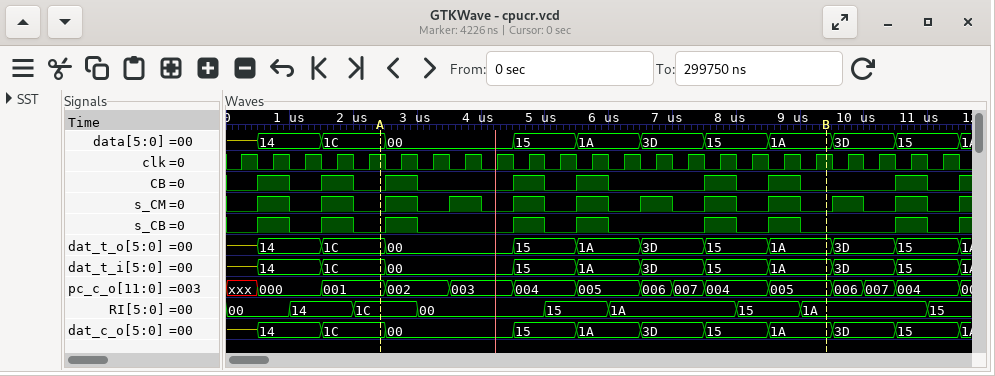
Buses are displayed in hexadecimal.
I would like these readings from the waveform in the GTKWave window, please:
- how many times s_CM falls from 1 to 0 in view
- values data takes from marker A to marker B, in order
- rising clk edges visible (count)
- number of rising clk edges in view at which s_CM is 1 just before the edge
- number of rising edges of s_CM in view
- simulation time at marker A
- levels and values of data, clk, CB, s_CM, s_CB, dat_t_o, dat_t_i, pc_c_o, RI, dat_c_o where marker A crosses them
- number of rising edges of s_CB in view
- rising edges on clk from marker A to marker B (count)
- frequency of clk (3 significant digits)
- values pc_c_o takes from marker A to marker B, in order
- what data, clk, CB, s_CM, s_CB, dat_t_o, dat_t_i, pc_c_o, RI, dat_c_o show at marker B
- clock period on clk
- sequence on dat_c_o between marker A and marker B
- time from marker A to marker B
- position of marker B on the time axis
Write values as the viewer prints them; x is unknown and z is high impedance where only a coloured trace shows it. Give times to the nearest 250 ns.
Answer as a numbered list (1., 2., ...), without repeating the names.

1. 11
2. 1C, 00, 15, 1A, 3D, 15, 1A
3. 23
4. 11
5. 12
6. 2500 ns
7. data=1C, clk=1, CB=0, s_CM=0, s_CB=0, dat_t_o=1C, dat_t_i=1C, pc_c_o=001, RI=1C, dat_c_o=1C
8. 9
9. 14
10. 2.00 MHz
11. 001, 002, 003, 004, 005, 006, 007, 004, 005
12. data=1A, clk=1, CB=0, s_CM=0, s_CB=0, dat_t_o=1A, dat_t_i=1A, pc_c_o=005, RI=1A, dat_c_o=1A
13. 500 ns
14. 1C, 00, 15, 1A, 3D, 15, 1A
15. 7000 ns
16. 9500 ns
